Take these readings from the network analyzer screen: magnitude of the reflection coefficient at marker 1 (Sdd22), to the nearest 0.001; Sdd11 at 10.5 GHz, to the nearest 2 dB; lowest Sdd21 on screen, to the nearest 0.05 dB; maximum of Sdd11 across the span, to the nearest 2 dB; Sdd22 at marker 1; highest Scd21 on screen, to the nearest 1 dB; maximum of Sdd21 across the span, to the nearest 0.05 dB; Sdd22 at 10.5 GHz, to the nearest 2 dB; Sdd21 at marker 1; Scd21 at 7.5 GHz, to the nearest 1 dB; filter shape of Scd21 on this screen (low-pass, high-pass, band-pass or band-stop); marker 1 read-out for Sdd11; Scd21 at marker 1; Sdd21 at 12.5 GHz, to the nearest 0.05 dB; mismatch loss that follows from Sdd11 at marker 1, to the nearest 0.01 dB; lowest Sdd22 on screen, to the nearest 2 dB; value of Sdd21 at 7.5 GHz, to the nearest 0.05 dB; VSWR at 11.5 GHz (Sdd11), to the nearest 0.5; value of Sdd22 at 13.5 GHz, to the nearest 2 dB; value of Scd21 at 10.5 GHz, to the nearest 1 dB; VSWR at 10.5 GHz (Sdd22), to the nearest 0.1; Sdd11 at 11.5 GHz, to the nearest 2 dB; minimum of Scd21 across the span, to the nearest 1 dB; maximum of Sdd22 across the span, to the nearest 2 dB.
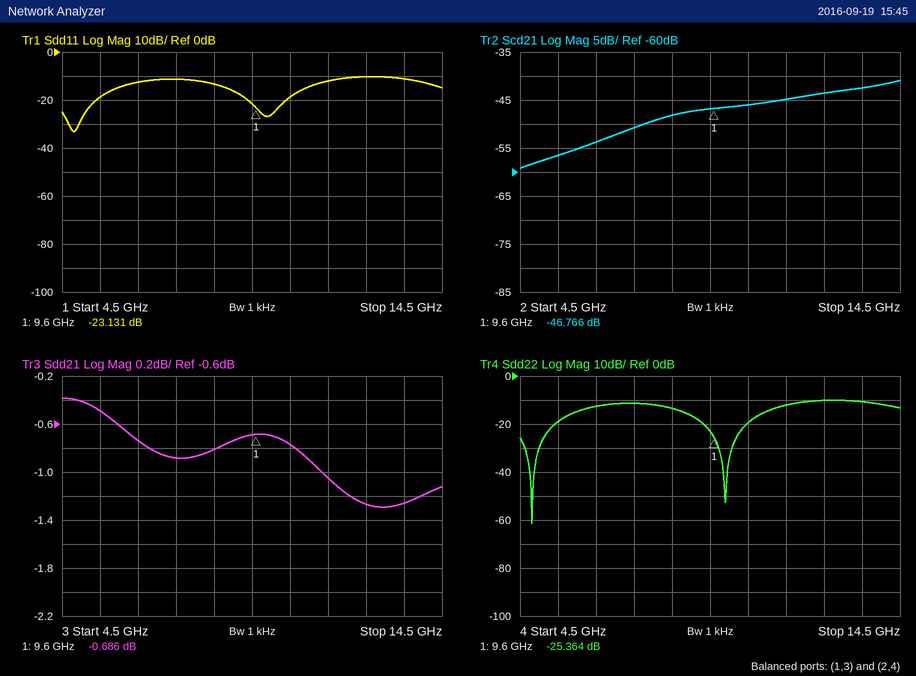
0.054
-18 dB
-1.30 dB
-10 dB
-25.364 dB
-41 dB
-0.40 dB
-20 dB
-0.686 dB
-51 dB
high-pass
-23.131 dB
-46.766 dB
-1.25 dB
0.02 dB
-62 dB
-0.90 dB
1.5
-10 dB
-46 dB
1.2
-12 dB
-59 dB
-10 dB
